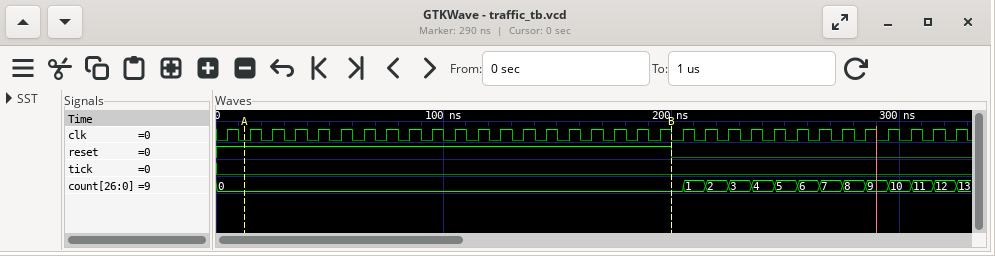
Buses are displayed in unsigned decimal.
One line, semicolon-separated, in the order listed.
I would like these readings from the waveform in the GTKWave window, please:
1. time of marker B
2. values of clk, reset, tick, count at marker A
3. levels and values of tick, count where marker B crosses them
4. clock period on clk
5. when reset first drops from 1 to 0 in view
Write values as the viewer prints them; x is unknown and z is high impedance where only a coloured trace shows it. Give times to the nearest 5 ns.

200 ns; clk=0, reset=1, tick=0, count=0; tick=0, count=0; 10 ns; 200 ns
